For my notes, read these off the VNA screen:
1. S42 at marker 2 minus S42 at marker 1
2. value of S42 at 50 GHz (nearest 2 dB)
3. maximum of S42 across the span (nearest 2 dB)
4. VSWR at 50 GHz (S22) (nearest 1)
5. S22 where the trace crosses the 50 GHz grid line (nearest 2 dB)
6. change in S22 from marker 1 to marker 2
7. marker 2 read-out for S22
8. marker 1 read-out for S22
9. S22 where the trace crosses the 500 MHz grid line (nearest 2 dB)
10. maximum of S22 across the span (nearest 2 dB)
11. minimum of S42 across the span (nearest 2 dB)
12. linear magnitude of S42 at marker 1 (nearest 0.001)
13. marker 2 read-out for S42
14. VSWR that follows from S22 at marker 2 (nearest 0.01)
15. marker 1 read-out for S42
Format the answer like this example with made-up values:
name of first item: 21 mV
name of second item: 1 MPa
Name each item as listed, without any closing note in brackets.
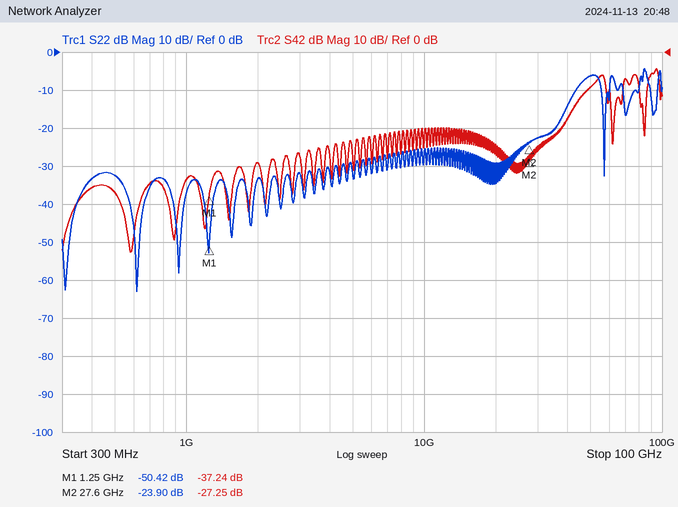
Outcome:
S42 at marker 2 minus S42 at marker 1: 9.99 dB
value of S42 at 50 GHz: -10 dB
maximum of S42 across the span: -4 dB
VSWR at 50 GHz (S22): 3
S22 where the trace crosses the 50 GHz grid line: -6 dB
change in S22 from marker 1 to marker 2: 26.52 dB
marker 2 read-out for S22: -23.90 dB
marker 1 read-out for S22: -50.42 dB
S22 where the trace crosses the 500 MHz grid line: -32 dB
maximum of S22 across the span: -4 dB
minimum of S42 across the span: -52 dB
linear magnitude of S42 at marker 1: 0.014
marker 2 read-out for S42: -27.25 dB
VSWR that follows from S22 at marker 2: 1.14
marker 1 read-out for S42: -37.24 dB
